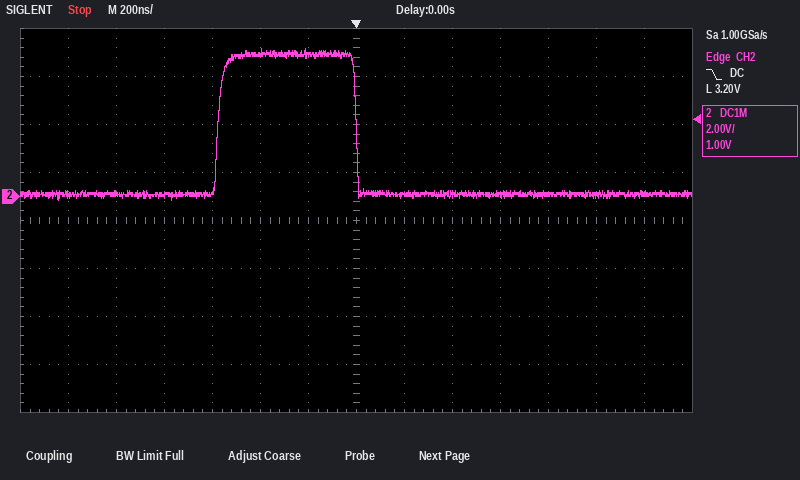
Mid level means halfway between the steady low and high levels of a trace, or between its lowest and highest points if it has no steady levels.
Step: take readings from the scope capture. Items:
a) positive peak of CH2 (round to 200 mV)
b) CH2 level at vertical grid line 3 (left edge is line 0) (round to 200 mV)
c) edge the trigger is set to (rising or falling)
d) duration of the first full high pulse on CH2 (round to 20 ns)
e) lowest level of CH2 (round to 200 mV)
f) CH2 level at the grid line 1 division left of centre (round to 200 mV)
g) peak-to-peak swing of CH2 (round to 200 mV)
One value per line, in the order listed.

6.2 V
0.0 V
falling
580 ns
-200 mV
5.8 V
6.4 V
